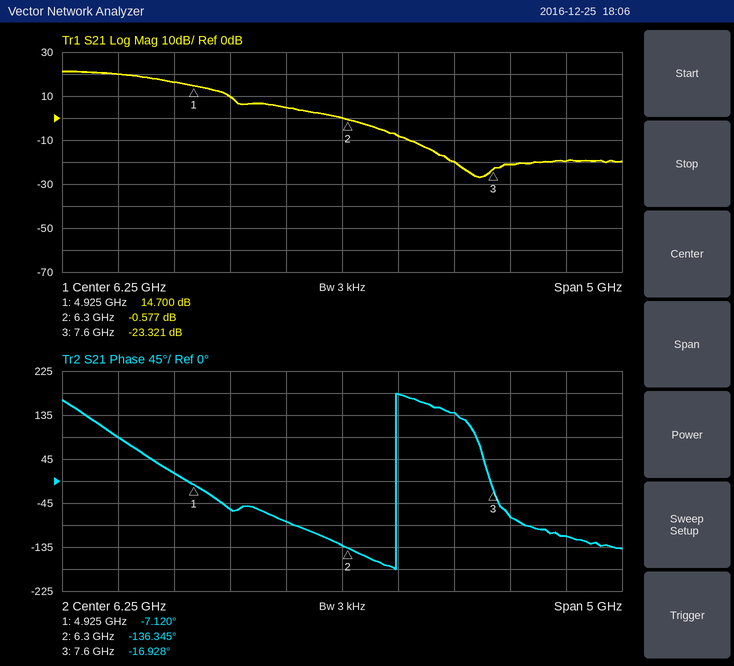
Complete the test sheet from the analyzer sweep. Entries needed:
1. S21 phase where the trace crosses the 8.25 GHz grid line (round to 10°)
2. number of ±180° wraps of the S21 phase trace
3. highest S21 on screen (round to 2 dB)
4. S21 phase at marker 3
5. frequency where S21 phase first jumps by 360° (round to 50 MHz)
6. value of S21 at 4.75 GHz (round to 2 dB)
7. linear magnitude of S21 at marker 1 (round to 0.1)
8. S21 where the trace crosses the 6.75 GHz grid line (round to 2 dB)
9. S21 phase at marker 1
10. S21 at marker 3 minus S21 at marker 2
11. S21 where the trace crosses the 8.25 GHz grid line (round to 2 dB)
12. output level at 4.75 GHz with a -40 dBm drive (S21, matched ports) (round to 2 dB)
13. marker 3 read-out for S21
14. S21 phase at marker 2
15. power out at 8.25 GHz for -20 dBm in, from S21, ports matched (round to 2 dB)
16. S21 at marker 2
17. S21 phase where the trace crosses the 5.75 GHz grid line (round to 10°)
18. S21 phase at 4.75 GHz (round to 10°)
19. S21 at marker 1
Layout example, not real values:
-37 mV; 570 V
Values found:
-110°; 1; 22 dB; -16.928°; 6.75 GHz; 16 dB; 5.4; -8 dB; -7.120°; -22.744 dB; -20 dB; -24 dBm; -23.321 dB; -136.345°; -40 dBm; -0.577 dB; -80°; 20°; 14.700 dB
